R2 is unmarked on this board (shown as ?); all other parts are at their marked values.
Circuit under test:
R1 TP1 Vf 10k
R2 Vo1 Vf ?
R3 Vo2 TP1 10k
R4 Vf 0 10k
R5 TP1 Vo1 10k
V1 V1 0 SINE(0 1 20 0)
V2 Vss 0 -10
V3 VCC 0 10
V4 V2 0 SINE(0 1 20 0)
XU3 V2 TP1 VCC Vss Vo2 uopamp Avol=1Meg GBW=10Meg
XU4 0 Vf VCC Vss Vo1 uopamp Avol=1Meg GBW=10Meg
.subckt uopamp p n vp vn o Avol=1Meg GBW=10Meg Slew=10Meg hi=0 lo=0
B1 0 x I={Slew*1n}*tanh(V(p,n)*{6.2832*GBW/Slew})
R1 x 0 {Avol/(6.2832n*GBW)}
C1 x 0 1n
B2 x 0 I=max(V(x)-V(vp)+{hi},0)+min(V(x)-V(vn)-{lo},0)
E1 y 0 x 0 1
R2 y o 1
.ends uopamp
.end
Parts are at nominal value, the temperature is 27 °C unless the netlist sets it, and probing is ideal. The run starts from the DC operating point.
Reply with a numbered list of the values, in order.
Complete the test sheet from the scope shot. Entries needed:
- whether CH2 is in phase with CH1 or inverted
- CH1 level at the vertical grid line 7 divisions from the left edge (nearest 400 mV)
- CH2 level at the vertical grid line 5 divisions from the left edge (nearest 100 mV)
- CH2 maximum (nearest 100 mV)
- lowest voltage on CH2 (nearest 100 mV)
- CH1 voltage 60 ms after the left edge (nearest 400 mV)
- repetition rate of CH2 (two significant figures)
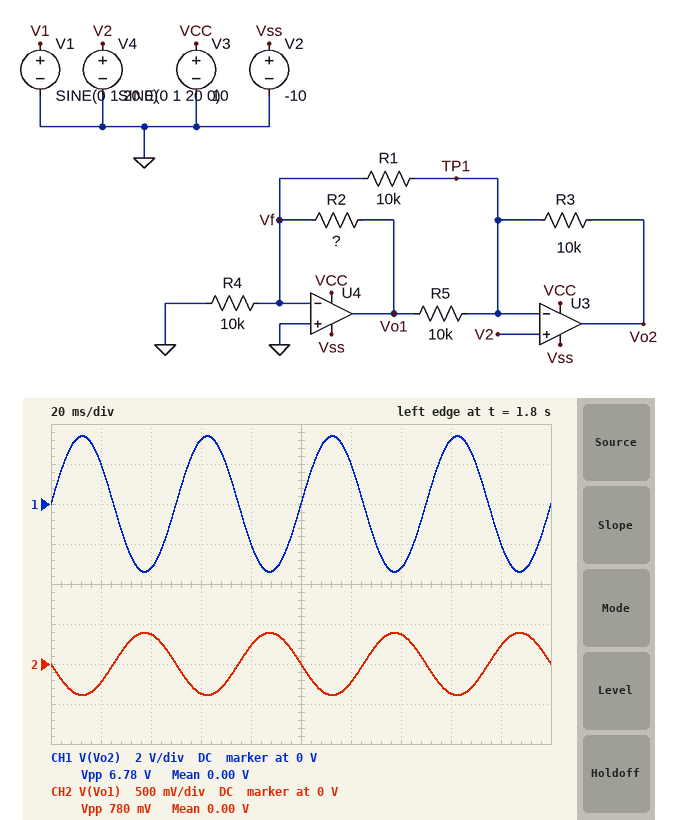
1. inverted
2. -3.2 V
3. 0 V
4. 400 mV
5. -400 mV
6. 3.2 V
7. 20 Hz
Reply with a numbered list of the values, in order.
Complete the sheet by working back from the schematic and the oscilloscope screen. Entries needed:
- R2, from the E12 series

1. 3.9 kΩ
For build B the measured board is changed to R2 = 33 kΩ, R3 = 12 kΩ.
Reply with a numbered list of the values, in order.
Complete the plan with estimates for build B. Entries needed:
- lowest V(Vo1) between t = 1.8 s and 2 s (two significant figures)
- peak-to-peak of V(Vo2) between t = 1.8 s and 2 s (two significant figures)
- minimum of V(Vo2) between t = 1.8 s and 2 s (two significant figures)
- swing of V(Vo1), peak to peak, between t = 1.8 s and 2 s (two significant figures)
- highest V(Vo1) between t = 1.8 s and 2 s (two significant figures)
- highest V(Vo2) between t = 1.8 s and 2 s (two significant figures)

1. -3.3 V
2. 15 V
3. -7.4 V
4. 6.6 V
5. 3.3 V
6. 7.4 V
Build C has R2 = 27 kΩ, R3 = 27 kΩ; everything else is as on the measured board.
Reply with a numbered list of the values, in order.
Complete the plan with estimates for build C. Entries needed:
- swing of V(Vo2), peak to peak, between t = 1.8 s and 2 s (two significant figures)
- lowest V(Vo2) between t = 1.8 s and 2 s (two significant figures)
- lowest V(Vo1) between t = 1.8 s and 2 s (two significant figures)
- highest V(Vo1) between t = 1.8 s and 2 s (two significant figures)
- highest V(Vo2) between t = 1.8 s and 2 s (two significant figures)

1. 20 V
2. -10 V
3. -2.0 V
4. 2.0 V
5. 10 V
